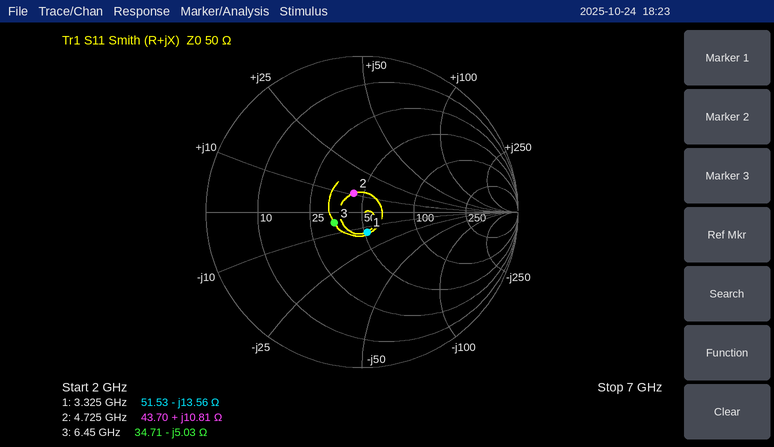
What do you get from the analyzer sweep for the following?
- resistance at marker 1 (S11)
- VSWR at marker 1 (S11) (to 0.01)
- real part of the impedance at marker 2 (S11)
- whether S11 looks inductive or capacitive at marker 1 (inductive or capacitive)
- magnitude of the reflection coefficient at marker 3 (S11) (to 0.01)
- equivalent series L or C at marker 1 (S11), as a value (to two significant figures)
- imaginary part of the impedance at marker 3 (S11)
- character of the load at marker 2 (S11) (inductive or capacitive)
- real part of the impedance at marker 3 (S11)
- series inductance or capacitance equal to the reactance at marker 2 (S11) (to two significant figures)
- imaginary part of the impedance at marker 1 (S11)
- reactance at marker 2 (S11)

51.53 Ω
1.31
43.70 Ω
capacitive
0.19
3.5 pF
-5.03 Ω
inductive
34.71 Ω
360 pH
-13.56 Ω
+10.81 Ω
